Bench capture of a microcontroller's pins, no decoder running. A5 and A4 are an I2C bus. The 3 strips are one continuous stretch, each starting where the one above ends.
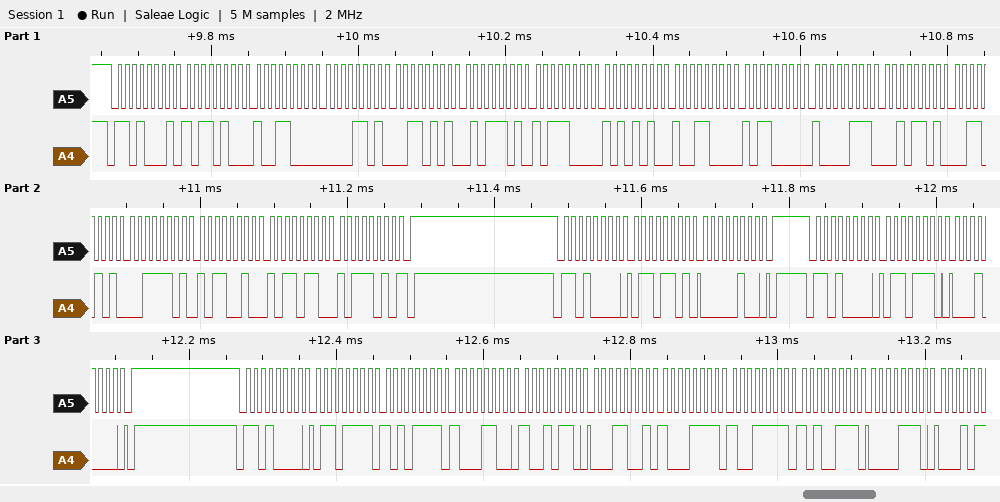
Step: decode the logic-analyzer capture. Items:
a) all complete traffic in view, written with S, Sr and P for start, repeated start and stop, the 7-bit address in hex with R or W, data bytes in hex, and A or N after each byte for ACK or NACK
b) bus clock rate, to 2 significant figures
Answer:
S 68R A B4 A 98 A 0D A 35 A 5D A B8 A AA A 98 A B0 A 87 A 2D A 35 A 3D A B2 A B6 A BA N P S 68W A 6D A 04 A P S 68W A 6E A 10 A P S 68W A 6F A AF A 8C A 96 A 19 A 8F A 9F A A7 A 0E A
100 kHz
